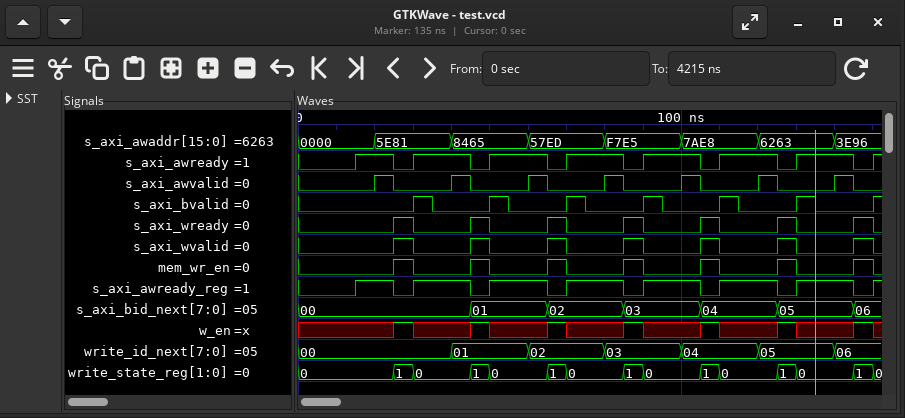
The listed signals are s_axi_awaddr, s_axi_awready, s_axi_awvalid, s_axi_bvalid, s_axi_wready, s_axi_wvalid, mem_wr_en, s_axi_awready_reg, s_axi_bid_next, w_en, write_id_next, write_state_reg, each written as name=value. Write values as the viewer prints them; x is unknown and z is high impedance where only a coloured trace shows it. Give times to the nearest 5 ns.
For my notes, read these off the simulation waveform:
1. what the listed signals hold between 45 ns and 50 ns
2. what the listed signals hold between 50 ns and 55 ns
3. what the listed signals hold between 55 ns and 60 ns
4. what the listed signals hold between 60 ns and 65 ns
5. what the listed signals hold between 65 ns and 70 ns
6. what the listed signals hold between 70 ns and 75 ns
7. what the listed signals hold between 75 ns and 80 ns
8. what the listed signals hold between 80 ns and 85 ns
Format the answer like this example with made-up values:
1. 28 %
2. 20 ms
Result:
1. s_axi_awaddr=8465, s_axi_awready=0, s_axi_awvalid=0, s_axi_bvalid=0, s_axi_wready=1, s_axi_wvalid=1, mem_wr_en=1, s_axi_awready_reg=0, s_axi_bid_next=01, w_en=1, write_id_next=01, write_state_reg=1
2. s_axi_awaddr=8465, s_axi_awready=1, s_axi_awvalid=0, s_axi_bvalid=1, s_axi_wready=0, s_axi_wvalid=0, mem_wr_en=0, s_axi_awready_reg=1, s_axi_bid_next=01, w_en=x, write_id_next=01, write_state_reg=0
3. s_axi_awaddr=8465, s_axi_awready=1, s_axi_awvalid=0, s_axi_bvalid=0, s_axi_wready=0, s_axi_wvalid=0, mem_wr_en=0, s_axi_awready_reg=1, s_axi_bid_next=01, w_en=x, write_id_next=01, write_state_reg=0
4. s_axi_awaddr=57ED, s_axi_awready=1, s_axi_awvalid=1, s_axi_bvalid=0, s_axi_wready=0, s_axi_wvalid=0, mem_wr_en=0, s_axi_awready_reg=1, s_axi_bid_next=01, w_en=x, write_id_next=02, write_state_reg=0
5. s_axi_awaddr=57ED, s_axi_awready=0, s_axi_awvalid=0, s_axi_bvalid=0, s_axi_wready=1, s_axi_wvalid=1, mem_wr_en=1, s_axi_awready_reg=0, s_axi_bid_next=02, w_en=1, write_id_next=02, write_state_reg=1
6. s_axi_awaddr=57ED, s_axi_awready=1, s_axi_awvalid=0, s_axi_bvalid=1, s_axi_wready=0, s_axi_wvalid=0, mem_wr_en=0, s_axi_awready_reg=1, s_axi_bid_next=02, w_en=x, write_id_next=02, write_state_reg=0
7. s_axi_awaddr=57ED, s_axi_awready=1, s_axi_awvalid=0, s_axi_bvalid=0, s_axi_wready=0, s_axi_wvalid=0, mem_wr_en=0, s_axi_awready_reg=1, s_axi_bid_next=02, w_en=x, write_id_next=02, write_state_reg=0
8. s_axi_awaddr=F7E5, s_axi_awready=1, s_axi_awvalid=1, s_axi_bvalid=0, s_axi_wready=0, s_axi_wvalid=0, mem_wr_en=0, s_axi_awready_reg=1, s_axi_bid_next=02, w_en=x, write_id_next=03, write_state_reg=0
